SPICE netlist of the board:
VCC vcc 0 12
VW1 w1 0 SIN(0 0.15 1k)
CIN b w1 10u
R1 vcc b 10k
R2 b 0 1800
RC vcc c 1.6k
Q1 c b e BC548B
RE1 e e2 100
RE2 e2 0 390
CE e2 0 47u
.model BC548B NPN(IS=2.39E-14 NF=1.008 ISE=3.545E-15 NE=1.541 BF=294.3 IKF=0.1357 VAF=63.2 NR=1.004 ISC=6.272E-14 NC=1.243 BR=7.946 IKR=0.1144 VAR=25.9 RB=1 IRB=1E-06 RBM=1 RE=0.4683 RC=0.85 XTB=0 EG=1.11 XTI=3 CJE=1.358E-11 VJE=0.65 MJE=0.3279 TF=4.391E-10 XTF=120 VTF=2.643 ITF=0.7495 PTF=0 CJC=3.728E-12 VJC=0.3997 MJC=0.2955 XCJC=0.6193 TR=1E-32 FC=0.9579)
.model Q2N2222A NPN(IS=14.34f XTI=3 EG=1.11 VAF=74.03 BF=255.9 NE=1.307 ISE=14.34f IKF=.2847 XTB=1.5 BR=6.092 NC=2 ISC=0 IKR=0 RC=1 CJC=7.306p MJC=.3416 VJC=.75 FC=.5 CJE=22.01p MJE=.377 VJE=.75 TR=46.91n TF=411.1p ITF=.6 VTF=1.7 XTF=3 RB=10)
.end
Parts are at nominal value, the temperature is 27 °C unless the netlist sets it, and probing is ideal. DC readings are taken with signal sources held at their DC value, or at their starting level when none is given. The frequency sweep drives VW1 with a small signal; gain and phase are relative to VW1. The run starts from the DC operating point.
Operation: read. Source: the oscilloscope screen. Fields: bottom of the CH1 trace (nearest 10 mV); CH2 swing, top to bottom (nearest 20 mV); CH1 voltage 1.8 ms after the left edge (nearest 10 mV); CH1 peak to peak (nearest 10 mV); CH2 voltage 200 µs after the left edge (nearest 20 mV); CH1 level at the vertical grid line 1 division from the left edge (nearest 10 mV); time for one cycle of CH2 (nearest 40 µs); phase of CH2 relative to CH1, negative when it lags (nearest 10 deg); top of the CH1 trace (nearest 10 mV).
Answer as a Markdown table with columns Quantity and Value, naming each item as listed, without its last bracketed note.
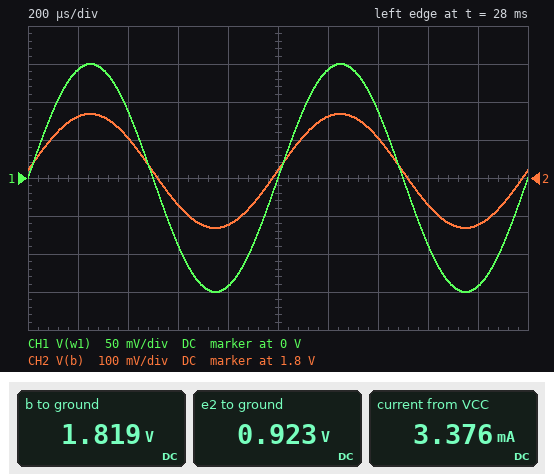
| Quantity | Value |
|---|---|
| bottom of the CH1 trace | -150 mV |
| CH2 swing, top to bottom | 300 mV |
| CH1 voltage 1.8 ms after the left edge | -140 mV |
| CH1 peak to peak | 300 mV |
| CH2 voltage 200 µs after the left edge | 1.96 V |
| CH1 level at the vertical grid line 1 division from the left edge | 140 mV |
| time for one cycle of CH2 | 1.00 ms |
| phase of CH2 relative to CH1, negative when it lags | 0 deg |
| top of the CH1 trace | 150 mV |
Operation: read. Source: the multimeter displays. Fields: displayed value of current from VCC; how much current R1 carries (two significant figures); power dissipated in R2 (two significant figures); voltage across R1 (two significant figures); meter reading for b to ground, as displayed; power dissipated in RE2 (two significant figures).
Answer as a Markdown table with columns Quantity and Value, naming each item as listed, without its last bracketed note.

| Quantity | Value |
|---|---|
| displayed value of current from VCC | 3.376 mA |
| how much current R1 carries | 1.0 mA |
| power dissipated in R2 | 1.8 mW |
| voltage across R1 | 10 V |
| meter reading for b to ground, as displayed | 1.819 V |
| power dissipated in RE2 | 2.2 mW |
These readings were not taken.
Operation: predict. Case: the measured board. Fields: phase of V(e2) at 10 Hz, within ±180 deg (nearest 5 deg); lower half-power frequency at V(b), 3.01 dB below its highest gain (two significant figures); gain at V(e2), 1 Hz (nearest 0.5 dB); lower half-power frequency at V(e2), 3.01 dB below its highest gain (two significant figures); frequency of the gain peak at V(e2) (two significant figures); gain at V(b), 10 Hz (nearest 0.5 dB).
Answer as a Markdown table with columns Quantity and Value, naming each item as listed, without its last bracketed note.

| Quantity | Value |
|---|---|
| phase of V(e2) at 10 Hz, within ±180 deg | 30 deg |
| lower half-power frequency at V(b), 3.01 dB below its highest gain | 11 Hz |
| gain at V(e2), 1 Hz | -22.5 dB |
| lower half-power frequency at V(e2), 3.01 dB below its highest gain | 7.2 Hz |
| frequency of the gain peak at V(e2) | 20 Hz |
| gain at V(b), 10 Hz | -3.5 dB |
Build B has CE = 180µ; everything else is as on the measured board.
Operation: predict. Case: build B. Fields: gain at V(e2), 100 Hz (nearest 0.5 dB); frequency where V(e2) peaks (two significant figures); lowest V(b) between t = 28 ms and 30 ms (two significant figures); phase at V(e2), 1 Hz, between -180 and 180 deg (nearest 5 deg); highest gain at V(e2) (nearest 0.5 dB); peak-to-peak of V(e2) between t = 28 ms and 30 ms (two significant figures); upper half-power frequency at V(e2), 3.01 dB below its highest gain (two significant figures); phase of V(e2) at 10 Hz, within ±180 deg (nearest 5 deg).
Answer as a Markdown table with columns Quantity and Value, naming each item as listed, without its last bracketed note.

| Quantity | Value |
|---|---|
| gain at V(e2), 100 Hz | -22.0 dB |
| frequency where V(e2) peaks | 10 Hz |
| lowest V(b) between t = 28 ms and 30 ms | 1.7 V |
| phase at V(e2), 1 Hz, between -180 and 180 deg | 80 deg |
| highest gain at V(e2) | -8.5 dB |
| peak-to-peak of V(e2) between t = 28 ms and 30 ms | 2.4 mV |
| upper half-power frequency at V(e2), 3.01 dB below its highest gain | 25 Hz |
| phase of V(e2) at 10 Hz, within ±180 deg | 0 deg |
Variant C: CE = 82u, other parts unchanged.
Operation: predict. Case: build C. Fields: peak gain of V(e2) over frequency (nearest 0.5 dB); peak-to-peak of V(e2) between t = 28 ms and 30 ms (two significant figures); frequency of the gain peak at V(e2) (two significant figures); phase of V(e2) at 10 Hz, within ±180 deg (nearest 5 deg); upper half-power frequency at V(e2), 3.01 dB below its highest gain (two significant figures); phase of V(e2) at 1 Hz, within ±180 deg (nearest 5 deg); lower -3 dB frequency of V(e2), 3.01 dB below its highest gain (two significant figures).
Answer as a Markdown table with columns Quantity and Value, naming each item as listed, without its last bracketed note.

| Quantity | Value |
|---|---|
| peak gain of V(e2) over frequency | -5.5 dB |
| peak-to-peak of V(e2) between t = 28 ms and 30 ms | 5.2 mV |
| frequency of the gain peak at V(e2) | 15 Hz |
| phase of V(e2) at 10 Hz, within ±180 deg | 20 deg |
| upper half-power frequency at V(e2), 3.01 dB below its highest gain | 39 Hz |
| phase of V(e2) at 1 Hz, within ±180 deg | 80 deg |
| lower -3 dB frequency of V(e2), 3.01 dB below its highest gain | 6.0 Hz |
